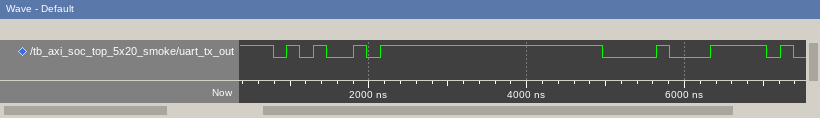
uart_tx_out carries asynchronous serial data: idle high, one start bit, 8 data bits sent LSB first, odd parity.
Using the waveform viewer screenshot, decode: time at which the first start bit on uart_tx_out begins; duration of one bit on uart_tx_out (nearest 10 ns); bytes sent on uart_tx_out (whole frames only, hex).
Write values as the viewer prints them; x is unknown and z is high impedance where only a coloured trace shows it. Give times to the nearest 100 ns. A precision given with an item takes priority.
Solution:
800 ns
170 ns
A5, 88
